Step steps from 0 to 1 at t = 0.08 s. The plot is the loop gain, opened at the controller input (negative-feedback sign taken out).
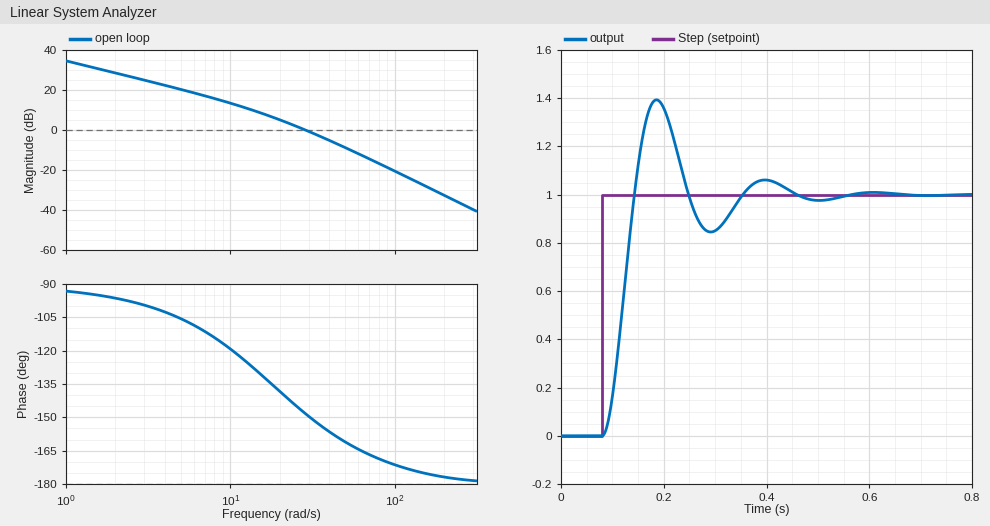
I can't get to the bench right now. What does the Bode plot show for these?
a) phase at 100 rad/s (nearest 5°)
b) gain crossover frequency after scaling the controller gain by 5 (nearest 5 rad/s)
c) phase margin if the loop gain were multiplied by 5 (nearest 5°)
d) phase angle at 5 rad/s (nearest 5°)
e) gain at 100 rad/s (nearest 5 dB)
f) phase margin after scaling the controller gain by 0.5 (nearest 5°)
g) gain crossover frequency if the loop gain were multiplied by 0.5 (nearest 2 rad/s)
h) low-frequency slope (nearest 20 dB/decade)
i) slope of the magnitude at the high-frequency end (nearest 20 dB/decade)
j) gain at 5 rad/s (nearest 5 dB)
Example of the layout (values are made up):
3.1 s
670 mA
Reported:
-170°
70 rad/s
15°
-105°
-20 dB
45°
18 rad/s
-20 dB/decade
-40 dB/decade
20 dB
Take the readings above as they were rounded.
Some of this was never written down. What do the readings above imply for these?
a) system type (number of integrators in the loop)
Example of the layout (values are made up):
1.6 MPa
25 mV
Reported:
1
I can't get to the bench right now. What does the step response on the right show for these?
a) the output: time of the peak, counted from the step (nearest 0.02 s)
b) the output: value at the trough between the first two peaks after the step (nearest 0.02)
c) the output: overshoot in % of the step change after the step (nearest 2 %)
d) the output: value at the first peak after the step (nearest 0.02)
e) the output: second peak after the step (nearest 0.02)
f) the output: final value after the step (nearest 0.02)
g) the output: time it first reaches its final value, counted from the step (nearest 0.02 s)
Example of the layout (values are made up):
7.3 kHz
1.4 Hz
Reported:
0.10 s
0.84
40 %
1.40
1.06
1.00
0.06 s
